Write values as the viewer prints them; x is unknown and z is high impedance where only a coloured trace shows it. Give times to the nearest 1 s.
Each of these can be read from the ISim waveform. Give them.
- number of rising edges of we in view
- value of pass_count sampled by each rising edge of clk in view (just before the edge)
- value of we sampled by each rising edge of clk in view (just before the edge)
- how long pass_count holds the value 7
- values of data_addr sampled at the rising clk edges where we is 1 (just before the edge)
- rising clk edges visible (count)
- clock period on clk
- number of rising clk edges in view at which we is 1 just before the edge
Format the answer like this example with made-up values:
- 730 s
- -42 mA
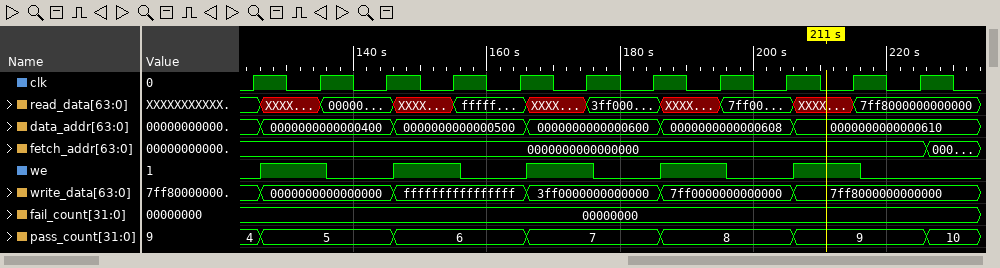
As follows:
- 5
- 4, 5, 5, 6, 6, 7, 7, 8, 8, 9, 9
- 0 1 0 1 0 1 0 1 0 1 0
- 20 s
- 0000000000000400, 0000000000000500, 0000000000000600, 0000000000000608, 0000000000000610
- 11
- 10 s
- 5
